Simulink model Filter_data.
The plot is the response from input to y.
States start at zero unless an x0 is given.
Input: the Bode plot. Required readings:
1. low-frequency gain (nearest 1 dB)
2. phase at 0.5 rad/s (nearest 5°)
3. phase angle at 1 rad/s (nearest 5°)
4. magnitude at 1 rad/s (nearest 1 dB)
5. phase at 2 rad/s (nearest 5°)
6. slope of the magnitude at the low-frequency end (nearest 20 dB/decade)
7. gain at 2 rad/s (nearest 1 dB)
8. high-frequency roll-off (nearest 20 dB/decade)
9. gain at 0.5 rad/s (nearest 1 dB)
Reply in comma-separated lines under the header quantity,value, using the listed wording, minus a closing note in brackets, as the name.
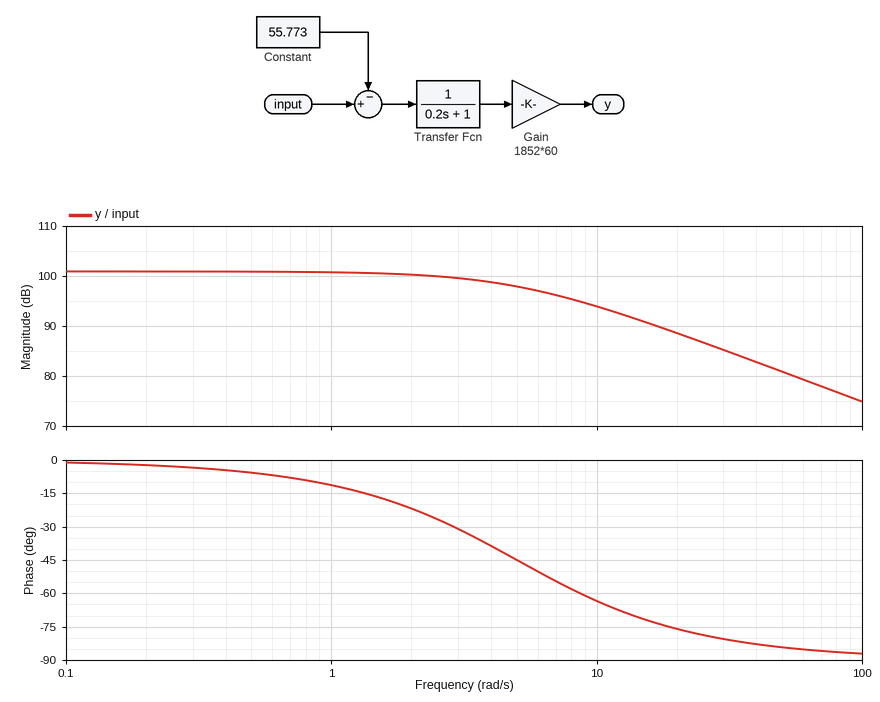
quantity,value
low-frequency gain,101 dB
phase at 0.5 rad/s,-5°
phase angle at 1 rad/s,-10°
magnitude at 1 rad/s,101 dB
phase at 2 rad/s,-20°
slope of the magnitude at the low-frequency end,0 dB/decade
gain at 2 rad/s,100 dB
high-frequency roll-off,-20 dB/decade
gain at 0.5 rad/s,101 dB
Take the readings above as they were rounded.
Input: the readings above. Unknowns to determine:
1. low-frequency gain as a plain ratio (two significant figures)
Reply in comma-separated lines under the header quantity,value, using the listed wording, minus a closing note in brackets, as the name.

quantity,value
low-frequency gain as a plain ratio,110000
